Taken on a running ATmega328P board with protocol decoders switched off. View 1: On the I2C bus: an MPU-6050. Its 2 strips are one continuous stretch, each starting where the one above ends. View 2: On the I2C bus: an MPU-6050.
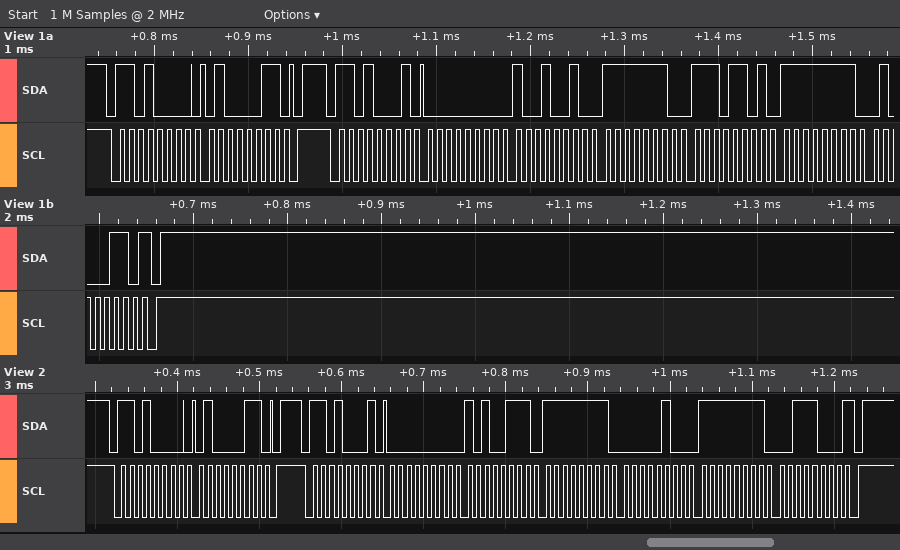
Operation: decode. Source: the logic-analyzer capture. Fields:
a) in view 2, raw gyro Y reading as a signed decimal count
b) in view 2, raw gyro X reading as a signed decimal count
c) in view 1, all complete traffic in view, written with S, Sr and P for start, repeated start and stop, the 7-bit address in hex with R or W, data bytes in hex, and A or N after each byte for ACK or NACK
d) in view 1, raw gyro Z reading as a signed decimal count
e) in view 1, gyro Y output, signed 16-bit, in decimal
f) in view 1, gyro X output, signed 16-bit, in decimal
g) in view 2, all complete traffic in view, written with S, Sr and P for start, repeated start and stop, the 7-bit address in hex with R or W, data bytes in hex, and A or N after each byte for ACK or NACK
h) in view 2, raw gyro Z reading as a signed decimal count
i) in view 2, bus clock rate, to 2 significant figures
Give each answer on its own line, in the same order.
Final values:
-252
167
S 68W A 43 A P S 68R A 00 A 92 A FE A ED A FF A 46 N P
-186
-275
146
S 68W A 43 A P S 68R A 00 A A7 A FF A 04 A FF A 38 N P
-200
100 kHz
